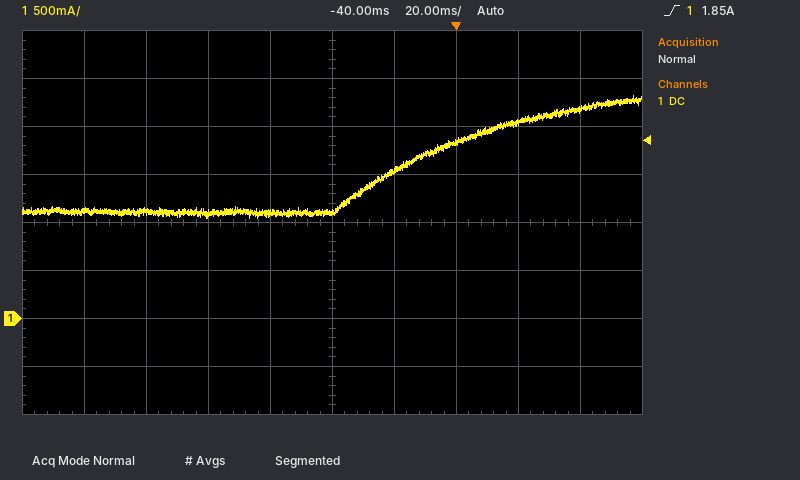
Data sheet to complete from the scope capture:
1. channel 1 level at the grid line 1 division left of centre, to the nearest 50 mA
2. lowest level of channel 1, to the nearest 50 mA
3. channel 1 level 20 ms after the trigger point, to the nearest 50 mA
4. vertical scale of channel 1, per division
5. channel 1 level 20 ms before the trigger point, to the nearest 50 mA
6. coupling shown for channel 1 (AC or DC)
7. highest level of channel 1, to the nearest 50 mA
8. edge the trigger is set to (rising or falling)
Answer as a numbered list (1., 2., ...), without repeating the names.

1. 1.10 A
2. 1.05 A
3. 2.05 A
4. 500 mA
5. 1.55 A
6. DC
7. 2.30 A
8. rising
